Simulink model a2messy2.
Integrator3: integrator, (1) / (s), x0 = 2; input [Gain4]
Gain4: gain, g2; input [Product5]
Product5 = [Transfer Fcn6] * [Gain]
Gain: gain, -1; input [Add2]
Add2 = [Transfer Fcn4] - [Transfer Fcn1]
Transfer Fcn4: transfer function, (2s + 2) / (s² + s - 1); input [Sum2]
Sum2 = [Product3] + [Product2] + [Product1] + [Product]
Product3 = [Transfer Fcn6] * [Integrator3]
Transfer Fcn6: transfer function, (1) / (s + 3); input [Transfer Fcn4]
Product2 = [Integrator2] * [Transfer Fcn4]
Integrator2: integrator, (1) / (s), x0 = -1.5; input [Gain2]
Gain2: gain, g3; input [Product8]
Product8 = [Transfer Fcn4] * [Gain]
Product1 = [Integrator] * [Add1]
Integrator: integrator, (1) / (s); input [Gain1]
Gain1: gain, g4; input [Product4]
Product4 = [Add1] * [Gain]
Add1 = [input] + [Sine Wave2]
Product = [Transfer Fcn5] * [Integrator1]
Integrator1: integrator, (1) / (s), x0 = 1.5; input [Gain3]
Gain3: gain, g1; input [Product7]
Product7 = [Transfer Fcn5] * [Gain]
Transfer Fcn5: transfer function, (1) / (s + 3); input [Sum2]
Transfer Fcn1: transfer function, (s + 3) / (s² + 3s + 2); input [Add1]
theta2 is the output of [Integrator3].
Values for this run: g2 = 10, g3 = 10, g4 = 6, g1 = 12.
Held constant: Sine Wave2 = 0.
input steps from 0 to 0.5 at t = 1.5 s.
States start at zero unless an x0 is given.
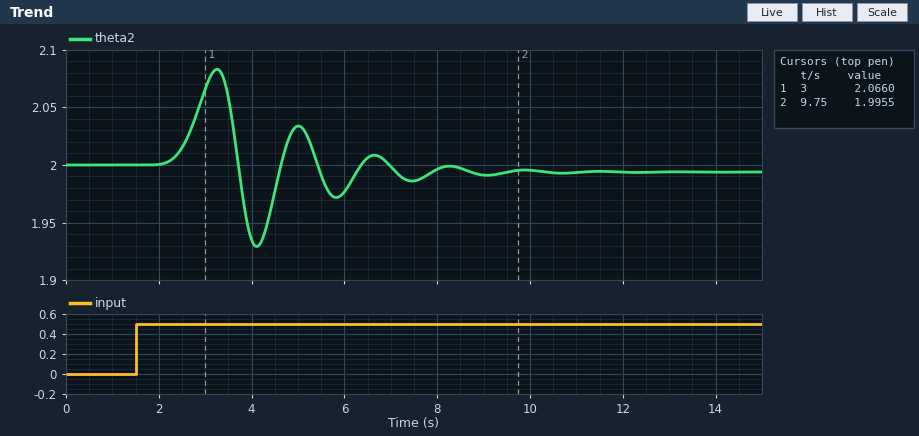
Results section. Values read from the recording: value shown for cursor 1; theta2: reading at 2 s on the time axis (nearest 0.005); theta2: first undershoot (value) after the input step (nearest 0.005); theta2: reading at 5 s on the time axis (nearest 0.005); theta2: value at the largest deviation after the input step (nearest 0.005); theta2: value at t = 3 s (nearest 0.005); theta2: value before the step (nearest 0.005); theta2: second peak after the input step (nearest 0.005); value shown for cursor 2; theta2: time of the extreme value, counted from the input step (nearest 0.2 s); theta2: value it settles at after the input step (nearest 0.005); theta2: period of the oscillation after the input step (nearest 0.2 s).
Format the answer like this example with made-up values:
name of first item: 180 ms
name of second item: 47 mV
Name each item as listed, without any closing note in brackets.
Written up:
value shown for cursor 1: 2.0660
theta2: reading at 2 s on the time axis: 2.000
theta2: first undershoot (value) after the input step: 1.930
theta2: reading at 5 s on the time axis: 2.035
theta2: value at the largest deviation after the input step: 2.085
theta2: value at t = 3 s: 2.065
theta2: value before the step: 2.000
theta2: second peak after the input step: 2.035
value shown for cursor 2: 1.9955
theta2: time of the extreme value, counted from the input step: 1.8 s
theta2: value it settles at after the input step: 1.995
theta2: period of the oscillation after the input step: 1.8 s
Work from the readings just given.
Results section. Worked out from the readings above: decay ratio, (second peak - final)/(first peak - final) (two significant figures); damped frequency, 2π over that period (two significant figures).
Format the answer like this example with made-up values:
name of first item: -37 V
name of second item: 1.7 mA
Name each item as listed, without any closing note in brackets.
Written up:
decay ratio, (second peak - final)/(first peak - final): 0.44
damped frequency, 2π over that period: 3.5 rad/s
